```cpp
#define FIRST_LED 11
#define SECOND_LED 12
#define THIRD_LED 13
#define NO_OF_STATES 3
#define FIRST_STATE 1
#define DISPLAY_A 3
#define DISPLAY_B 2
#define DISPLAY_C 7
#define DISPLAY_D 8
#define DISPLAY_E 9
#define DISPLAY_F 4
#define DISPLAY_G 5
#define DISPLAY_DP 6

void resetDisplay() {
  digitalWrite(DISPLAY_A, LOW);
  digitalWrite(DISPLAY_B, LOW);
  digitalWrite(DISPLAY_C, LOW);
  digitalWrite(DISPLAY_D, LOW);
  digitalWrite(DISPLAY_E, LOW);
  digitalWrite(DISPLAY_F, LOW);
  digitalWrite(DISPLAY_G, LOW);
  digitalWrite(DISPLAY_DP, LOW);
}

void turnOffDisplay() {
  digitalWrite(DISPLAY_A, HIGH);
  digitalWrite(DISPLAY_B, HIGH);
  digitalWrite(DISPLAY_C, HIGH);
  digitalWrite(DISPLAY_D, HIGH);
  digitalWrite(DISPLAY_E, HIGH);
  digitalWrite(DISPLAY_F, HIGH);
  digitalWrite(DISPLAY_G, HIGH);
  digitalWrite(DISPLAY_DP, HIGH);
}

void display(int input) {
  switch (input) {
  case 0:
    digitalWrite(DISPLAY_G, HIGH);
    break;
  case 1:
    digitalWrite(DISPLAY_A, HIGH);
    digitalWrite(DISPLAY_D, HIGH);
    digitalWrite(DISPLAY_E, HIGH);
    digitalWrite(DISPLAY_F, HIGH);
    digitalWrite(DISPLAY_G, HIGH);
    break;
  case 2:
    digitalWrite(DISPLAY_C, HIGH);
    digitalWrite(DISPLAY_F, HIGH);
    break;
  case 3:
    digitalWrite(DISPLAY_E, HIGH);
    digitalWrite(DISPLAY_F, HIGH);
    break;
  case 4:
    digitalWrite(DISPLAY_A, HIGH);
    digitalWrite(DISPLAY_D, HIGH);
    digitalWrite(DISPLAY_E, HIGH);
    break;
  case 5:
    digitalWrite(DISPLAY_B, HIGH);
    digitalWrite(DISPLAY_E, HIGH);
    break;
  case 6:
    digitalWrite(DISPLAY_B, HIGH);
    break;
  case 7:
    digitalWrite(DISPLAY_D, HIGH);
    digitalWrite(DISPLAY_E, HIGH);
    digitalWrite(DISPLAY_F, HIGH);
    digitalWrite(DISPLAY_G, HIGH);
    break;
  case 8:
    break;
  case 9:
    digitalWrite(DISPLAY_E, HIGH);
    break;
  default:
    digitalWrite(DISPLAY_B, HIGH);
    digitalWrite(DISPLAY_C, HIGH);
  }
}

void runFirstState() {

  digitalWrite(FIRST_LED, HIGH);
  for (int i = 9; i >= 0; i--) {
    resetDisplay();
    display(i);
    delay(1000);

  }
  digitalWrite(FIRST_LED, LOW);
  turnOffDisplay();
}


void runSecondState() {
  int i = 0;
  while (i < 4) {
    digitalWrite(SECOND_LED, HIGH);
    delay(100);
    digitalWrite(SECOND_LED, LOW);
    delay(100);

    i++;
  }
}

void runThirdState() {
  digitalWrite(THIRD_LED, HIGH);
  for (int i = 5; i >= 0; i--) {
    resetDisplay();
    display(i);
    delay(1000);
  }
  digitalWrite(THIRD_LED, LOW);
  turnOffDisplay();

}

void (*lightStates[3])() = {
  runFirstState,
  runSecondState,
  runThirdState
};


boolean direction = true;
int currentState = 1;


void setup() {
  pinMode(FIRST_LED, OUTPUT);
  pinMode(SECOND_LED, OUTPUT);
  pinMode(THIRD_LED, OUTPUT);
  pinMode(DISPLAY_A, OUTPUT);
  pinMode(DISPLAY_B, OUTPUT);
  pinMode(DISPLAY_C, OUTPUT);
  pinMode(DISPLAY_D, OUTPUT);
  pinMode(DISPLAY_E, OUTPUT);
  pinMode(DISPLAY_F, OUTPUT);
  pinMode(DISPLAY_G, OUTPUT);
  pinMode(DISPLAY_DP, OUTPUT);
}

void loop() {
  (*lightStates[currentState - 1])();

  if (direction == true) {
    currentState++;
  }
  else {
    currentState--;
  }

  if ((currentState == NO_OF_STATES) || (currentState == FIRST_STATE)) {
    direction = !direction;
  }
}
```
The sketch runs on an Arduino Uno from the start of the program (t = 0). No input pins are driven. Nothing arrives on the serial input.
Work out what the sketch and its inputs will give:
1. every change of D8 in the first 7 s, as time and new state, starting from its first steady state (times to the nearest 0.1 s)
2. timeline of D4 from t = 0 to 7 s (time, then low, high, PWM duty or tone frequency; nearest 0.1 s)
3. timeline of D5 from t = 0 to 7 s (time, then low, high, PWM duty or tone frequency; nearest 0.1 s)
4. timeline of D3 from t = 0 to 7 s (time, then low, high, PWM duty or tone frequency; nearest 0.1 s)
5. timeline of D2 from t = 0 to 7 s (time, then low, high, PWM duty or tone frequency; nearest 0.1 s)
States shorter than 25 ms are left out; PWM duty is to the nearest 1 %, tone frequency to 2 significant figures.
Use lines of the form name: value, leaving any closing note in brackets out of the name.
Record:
every change of D8 in the first 7 s, as time and new state, starting from its first steady state: 0 s low; 2 s high; 3 s low; 5 s high; 6 s low
timeline of D4 from t = 0 to 7 s: 0 s low; 2 s high; 3 s low; 6 s high
timeline of D5 from t = 0 to 7 s: 0 s low; 2 s high; 3 s low
timeline of D3 from t = 0 to 7 s: 0 s low; 5 s high; 6 s low
timeline of D2 from t = 0 to 7 s: 0 s low; 3 s high; 5 s low
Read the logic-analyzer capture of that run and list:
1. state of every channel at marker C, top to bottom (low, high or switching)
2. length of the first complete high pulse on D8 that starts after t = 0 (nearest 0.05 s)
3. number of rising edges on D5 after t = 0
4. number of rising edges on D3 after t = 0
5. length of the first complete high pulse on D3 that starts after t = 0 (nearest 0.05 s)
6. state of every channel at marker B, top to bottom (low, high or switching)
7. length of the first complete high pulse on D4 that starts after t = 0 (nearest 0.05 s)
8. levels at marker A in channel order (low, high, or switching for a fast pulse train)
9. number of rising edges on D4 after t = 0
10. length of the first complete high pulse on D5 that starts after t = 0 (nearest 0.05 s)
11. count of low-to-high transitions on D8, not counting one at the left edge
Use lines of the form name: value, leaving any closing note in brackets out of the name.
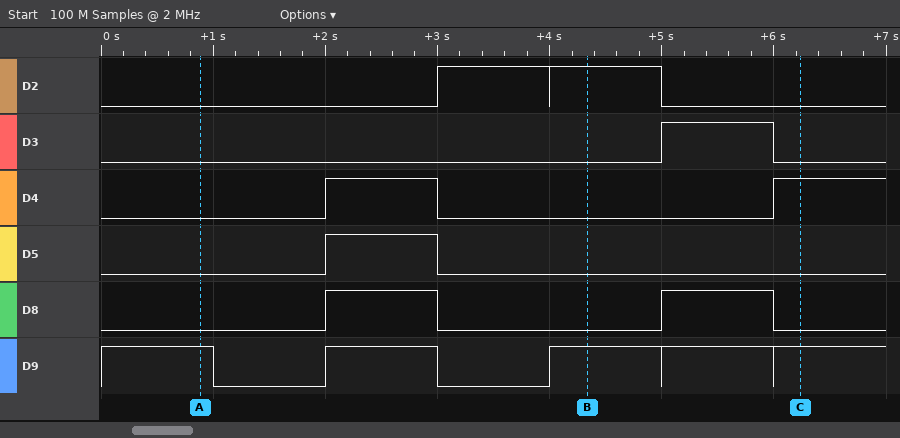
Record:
state of every channel at marker C, top to bottom: D2 low, D3 low, D4 high, D5 low, D8 low, D9 high
length of the first complete high pulse on D8 that starts after t = 0: 1.00 s
number of rising edges on D5 after t = 0: 1
number of rising edges on D3 after t = 0: 1
length of the first complete high pulse on D3 that starts after t = 0: 1.00 s
state of every channel at marker B, top to bottom: D2 high, D3 low, D4 low, D5 low, D8 low, D9 high
length of the first complete high pulse on D4 that starts after t = 0: 1.00 s
levels at marker A in channel order: D2 low, D3 low, D4 low, D5 low, D8 low, D9 high
number of rising edges on D4 after t = 0: 2
length of the first complete high pulse on D5 that starts after t = 0: 1.00 s
count of low-to-high transitions on D8, not counting one at the left edge: 2
